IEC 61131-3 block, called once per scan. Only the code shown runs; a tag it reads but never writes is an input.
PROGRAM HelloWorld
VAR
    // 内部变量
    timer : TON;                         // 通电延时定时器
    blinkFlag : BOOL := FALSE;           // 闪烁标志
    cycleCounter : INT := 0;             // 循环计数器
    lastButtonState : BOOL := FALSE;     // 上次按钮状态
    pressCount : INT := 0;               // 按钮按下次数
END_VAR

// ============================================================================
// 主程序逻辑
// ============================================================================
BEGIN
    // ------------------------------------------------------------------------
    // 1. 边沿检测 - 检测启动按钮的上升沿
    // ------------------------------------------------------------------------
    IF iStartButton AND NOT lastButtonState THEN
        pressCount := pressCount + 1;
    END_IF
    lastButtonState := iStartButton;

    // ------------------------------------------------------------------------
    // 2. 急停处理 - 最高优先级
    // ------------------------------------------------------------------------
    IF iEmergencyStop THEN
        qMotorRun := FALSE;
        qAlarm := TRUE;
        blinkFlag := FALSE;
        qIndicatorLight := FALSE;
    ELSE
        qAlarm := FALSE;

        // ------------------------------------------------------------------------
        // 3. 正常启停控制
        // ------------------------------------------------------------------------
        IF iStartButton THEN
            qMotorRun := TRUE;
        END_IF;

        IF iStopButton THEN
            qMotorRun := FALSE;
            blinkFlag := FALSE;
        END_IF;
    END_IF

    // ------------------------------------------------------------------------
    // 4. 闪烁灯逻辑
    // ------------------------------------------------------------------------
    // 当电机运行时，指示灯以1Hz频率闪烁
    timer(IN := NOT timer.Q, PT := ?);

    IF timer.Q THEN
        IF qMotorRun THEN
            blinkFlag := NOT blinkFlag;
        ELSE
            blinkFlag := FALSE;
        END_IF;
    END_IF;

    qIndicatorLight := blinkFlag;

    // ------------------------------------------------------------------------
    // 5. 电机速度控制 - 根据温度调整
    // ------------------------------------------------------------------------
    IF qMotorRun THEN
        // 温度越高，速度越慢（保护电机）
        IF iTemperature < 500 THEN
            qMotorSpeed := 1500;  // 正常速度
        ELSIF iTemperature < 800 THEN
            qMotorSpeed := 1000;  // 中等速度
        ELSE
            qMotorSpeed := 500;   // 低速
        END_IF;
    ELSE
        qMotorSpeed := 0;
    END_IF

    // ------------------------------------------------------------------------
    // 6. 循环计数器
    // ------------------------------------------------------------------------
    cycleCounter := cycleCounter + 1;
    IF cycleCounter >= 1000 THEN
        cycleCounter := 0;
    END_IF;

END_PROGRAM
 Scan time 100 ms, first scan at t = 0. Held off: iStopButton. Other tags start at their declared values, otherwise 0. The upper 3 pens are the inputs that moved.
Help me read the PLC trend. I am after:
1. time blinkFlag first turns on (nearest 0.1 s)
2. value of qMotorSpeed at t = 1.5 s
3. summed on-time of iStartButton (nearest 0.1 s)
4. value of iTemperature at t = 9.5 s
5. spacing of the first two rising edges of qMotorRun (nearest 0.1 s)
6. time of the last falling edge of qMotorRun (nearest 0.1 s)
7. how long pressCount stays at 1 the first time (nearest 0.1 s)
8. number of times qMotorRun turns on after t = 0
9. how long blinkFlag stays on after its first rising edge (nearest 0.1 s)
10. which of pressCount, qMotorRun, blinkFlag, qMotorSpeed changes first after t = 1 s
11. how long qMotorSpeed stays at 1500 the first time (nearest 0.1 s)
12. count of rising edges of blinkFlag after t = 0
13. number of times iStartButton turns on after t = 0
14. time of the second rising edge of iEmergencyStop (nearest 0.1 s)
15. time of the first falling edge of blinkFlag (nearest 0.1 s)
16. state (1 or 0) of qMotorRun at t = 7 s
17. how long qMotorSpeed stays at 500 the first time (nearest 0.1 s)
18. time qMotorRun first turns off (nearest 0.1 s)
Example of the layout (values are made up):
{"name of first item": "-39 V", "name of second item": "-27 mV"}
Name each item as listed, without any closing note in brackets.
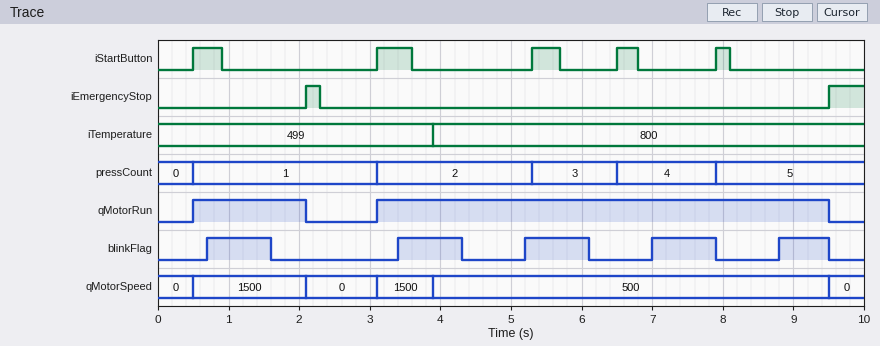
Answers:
{"time blinkFlag first turns on": "0.7 s", "value of qMotorSpeed at t = 1.5 s": "1500", "summed on-time of iStartButton": "1.8 s", "value of iTemperature at t = 9.5 s": "800", "spacing of the first two rising edges of qMotorRun": "2.6 s", "time of the last falling edge of qMotorRun": "9.5 s", "how long pressCount stays at 1 the first time": "2.6 s", "number of times qMotorRun turns on after t = 0": "2", "how long blinkFlag stays on after its first rising edge": "0.9 s", "which of pressCount, qMotorRun, blinkFlag, qMotorSpeed changes first after t = 1 s": "blinkFlag", "how long qMotorSpeed stays at 1500 the first time": "1.6 s", "count of rising edges of blinkFlag after t = 0": "5", "number of times iStartButton turns on after t = 0": "5", "time of the second rising edge of iEmergencyStop": "9.5 s", "time of the first falling edge of blinkFlag": "1.6 s", "state (1 or 0) of qMotorRun at t = 7 s": "1", "how long qMotorSpeed stays at 500 the first time": "5.6 s", "time qMotorRun first turns off": "2.1 s"}
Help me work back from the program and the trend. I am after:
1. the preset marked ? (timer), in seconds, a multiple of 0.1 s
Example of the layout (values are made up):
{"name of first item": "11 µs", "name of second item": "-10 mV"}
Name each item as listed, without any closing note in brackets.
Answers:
{"the preset marked ? (timer), in seconds, a multiple of 0.1 s": "0.7 s"}
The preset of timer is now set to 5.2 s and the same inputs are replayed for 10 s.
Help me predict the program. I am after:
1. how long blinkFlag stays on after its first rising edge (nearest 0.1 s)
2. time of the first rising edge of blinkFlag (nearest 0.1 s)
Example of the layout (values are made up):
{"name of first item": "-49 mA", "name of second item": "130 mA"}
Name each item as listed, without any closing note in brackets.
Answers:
{"how long blinkFlag stays on after its first rising edge": "4.3 s", "time of the first rising edge of blinkFlag": "5.2 s"}
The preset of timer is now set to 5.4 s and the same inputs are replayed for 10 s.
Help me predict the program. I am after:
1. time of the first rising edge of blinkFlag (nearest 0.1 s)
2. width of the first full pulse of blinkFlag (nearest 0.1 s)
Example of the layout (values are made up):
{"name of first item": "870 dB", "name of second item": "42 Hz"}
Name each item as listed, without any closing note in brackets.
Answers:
{"time of the first rising edge of blinkFlag": "5.4 s", "width of the first full pulse of blinkFlag": "4.1 s"}
